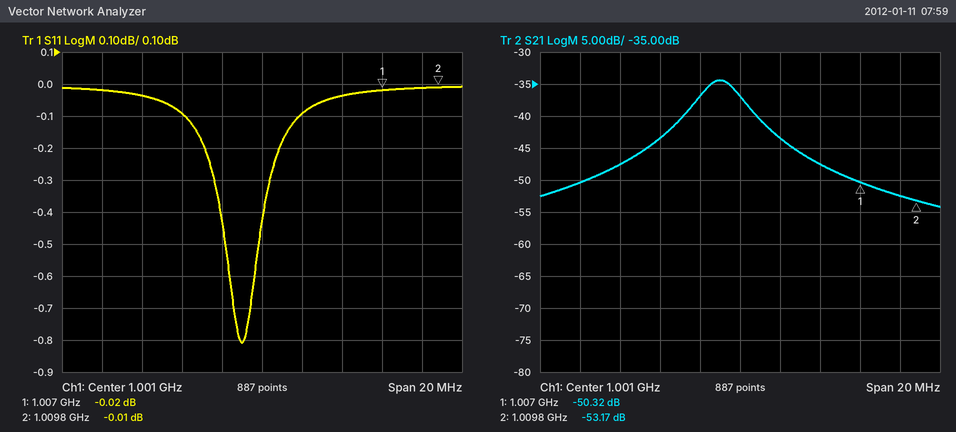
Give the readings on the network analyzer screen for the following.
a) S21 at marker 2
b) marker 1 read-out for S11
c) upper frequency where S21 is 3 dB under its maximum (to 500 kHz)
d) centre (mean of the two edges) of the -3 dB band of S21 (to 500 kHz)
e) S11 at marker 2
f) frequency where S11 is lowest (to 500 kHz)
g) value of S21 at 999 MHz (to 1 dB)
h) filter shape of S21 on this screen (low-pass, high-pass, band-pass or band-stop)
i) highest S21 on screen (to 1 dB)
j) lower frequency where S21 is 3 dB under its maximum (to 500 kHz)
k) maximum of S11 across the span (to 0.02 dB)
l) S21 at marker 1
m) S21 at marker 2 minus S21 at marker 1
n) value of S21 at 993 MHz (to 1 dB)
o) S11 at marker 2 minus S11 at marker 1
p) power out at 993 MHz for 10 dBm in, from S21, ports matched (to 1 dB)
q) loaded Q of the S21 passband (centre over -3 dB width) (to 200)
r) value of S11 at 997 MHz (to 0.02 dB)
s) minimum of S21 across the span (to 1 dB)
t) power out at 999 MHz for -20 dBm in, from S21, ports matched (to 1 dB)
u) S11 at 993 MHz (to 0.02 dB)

-53.17 dB
-0.02 dB
1.0010 GHz
1.0000 GHz
-0.01 dB
1.0000 GHz
-37 dB
band-pass
-34 dB
999.0 MHz
0.00 dB
-50.32 dB
-2.85 dB
-50 dB
0.01 dB
-40 dBm
400
-0.10 dB
-54 dB
-57 dBm
-0.02 dB
